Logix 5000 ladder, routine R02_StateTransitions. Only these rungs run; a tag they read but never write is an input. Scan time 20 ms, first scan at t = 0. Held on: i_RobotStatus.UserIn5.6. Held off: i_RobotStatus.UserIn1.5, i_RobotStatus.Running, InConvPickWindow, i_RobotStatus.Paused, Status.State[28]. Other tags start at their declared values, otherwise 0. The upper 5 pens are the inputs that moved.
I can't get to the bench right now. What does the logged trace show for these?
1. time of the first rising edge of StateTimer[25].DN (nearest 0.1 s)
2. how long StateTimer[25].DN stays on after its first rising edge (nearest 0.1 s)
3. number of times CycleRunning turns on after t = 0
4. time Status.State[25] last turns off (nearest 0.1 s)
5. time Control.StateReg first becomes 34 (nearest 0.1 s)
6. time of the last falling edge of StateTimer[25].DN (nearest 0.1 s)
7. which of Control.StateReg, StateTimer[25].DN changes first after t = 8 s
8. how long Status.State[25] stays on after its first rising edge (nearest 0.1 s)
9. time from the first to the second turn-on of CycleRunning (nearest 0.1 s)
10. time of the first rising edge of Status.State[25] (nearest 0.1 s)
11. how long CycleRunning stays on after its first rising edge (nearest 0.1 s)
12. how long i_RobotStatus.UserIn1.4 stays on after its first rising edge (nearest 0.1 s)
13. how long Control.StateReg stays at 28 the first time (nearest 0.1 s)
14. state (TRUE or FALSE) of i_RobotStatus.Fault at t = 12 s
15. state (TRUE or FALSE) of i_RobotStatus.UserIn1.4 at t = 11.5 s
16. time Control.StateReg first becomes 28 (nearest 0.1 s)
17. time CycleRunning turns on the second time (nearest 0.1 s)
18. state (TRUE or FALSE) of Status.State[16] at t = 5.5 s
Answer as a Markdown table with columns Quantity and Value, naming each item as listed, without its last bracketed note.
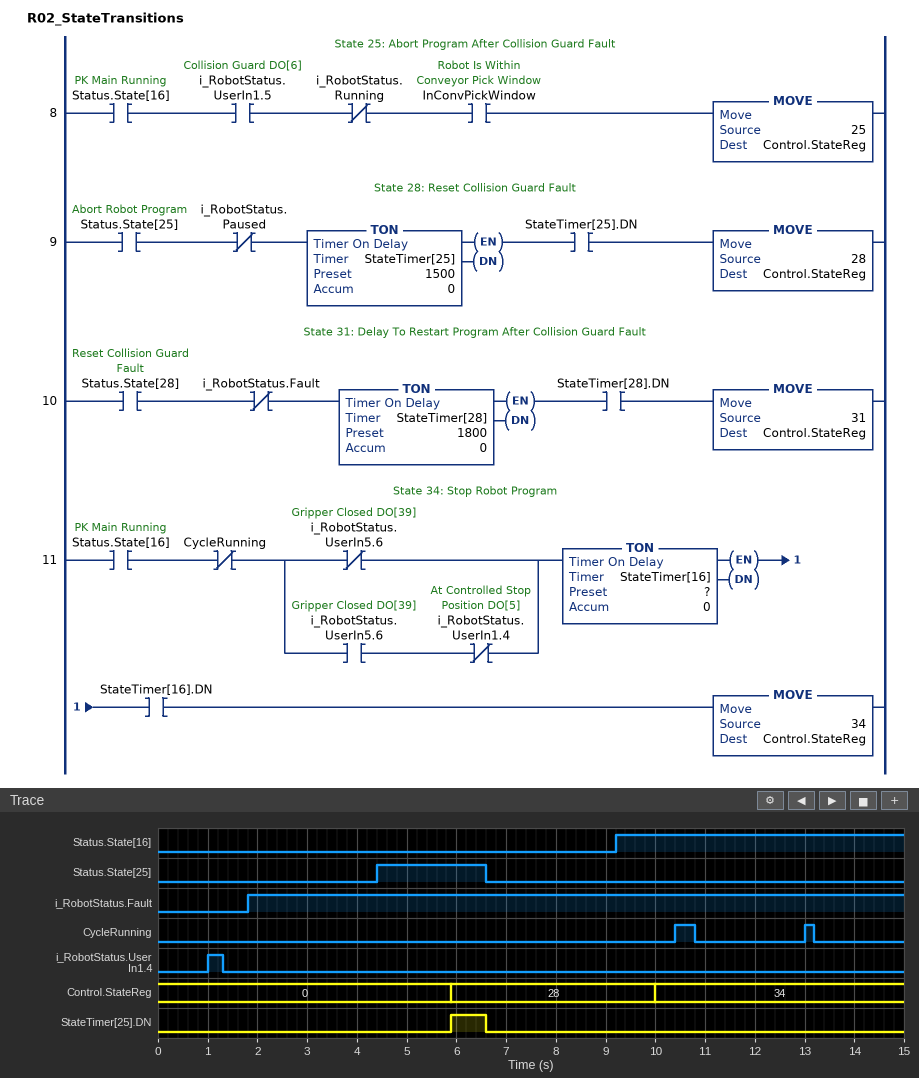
| Quantity | Value |
|---|---|
| time of the first rising edge of StateTimer[25].DN | 5.9 s |
| how long StateTimer[25].DN stays on after its first rising edge | 0.7 s |
| number of times CycleRunning turns on after t = 0 | 2 |
| time Status.State[25] last turns off | 6.6 s |
| time Control.StateReg first becomes 34 | 10.0 s |
| time of the last falling edge of StateTimer[25].DN | 6.6 s |
| which of Control.StateReg, StateTimer[25].DN changes first after t = 8 s | Control.StateReg |
| how long Status.State[25] stays on after its first rising edge | 2.2 s |
| time from the first to the second turn-on of CycleRunning | 2.6 s |
| time of the first rising edge of Status.State[25] | 4.4 s |
| how long CycleRunning stays on after its first rising edge | 0.4 s |
| how long i_RobotStatus.UserIn1.4 stays on after its first rising edge | 0.3 s |
| how long Control.StateReg stays at 28 the first time | 4.1 s |
| state (TRUE or FALSE) of i_RobotStatus.Fault at t = 12 s | TRUE |
| state (TRUE or FALSE) of i_RobotStatus.UserIn1.4 at t = 11.5 s | FALSE |
| time Control.StateReg first becomes 28 | 5.9 s |
| time CycleRunning turns on the second time | 13.0 s |
| state (TRUE or FALSE) of Status.State[16] at t = 5.5 s | FALSE |
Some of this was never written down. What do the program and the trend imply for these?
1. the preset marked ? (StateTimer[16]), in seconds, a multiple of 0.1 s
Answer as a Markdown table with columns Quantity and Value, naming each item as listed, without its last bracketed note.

| Quantity | Value |
|---|---|
| the preset marked ? (StateTimer[16]), in seconds, a multiple of 0.1 s | 0.8 s |
